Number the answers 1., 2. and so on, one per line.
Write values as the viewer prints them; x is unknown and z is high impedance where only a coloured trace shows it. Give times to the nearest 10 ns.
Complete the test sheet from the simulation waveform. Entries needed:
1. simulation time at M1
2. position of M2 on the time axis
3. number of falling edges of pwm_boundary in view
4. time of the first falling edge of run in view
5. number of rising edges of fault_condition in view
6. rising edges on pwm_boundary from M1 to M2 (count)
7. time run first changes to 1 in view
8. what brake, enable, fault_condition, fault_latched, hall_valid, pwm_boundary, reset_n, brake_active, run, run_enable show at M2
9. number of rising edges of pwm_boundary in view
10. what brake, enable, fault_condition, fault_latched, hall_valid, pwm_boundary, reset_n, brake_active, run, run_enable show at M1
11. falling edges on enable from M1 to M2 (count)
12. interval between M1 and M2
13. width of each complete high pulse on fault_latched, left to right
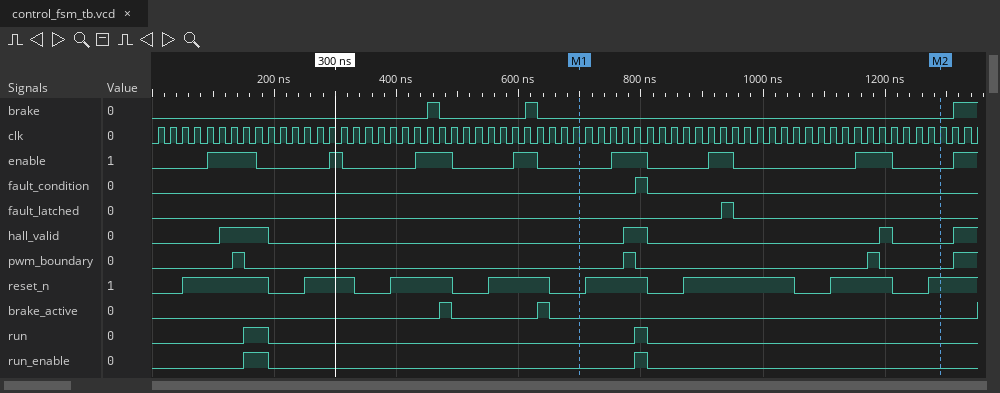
1. 700 ns
2. 1290 ns
3. 3
4. 190 ns
5. 1
6. 2
7. 150 ns
8. brake=0, enable=0, fault_condition=0, fault_latched=0, hall_valid=0, pwm_boundary=0, reset_n=1, brake_active=0, run=0, run_enable=0
9. 4
10. brake=0, enable=0, fault_condition=0, fault_latched=0, hall_valid=0, pwm_boundary=0, reset_n=0, brake_active=0, run=0, run_enable=0
11. 3
12. 590 ns
13. 20 ns
